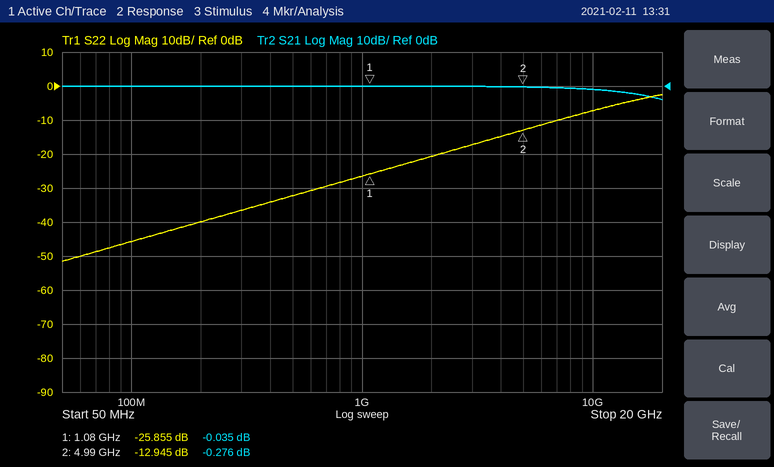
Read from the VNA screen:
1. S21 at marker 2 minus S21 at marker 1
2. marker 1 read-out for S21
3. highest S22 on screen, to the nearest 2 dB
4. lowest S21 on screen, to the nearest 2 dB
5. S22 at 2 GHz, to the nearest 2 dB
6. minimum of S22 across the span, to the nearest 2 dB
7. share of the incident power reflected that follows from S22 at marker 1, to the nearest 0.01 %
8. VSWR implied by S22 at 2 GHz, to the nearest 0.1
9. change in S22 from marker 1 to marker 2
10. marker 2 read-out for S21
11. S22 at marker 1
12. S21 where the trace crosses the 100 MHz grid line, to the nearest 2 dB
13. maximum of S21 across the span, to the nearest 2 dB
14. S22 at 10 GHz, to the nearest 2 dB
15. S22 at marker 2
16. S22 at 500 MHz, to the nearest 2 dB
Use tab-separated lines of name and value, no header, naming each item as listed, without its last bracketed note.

S21 at marker 2 minus S21 at marker 1	-0.241 dB
marker 1 read-out for S21	-0.035 dB
highest S22 on screen, to the nearest 2 dB	-2 dB
lowest S21 on screen, to the nearest 2 dB	-4 dB
S22 at 2 GHz, to the nearest 2 dB	-20 dB
minimum of S22 across the span, to the nearest 2 dB	-52 dB
share of the incident power reflected that follows from S22 at marker 1, to the nearest 0.01 %	0.26 %
VSWR implied by S22 at 2 GHz, to the nearest 0.1	1.2
change in S22 from marker 1 to marker 2	12.910 dB
marker 2 read-out for S21	-0.276 dB
S22 at marker 1	-25.855 dB
S21 where the trace crosses the 100 MHz grid line, to the nearest 2 dB	0 dB
maximum of S21 across the span, to the nearest 2 dB	0 dB
S22 at 10 GHz, to the nearest 2 dB	-8 dB
S22 at marker 2	-12.945 dB
S22 at 500 MHz, to the nearest 2 dB	-32 dB
